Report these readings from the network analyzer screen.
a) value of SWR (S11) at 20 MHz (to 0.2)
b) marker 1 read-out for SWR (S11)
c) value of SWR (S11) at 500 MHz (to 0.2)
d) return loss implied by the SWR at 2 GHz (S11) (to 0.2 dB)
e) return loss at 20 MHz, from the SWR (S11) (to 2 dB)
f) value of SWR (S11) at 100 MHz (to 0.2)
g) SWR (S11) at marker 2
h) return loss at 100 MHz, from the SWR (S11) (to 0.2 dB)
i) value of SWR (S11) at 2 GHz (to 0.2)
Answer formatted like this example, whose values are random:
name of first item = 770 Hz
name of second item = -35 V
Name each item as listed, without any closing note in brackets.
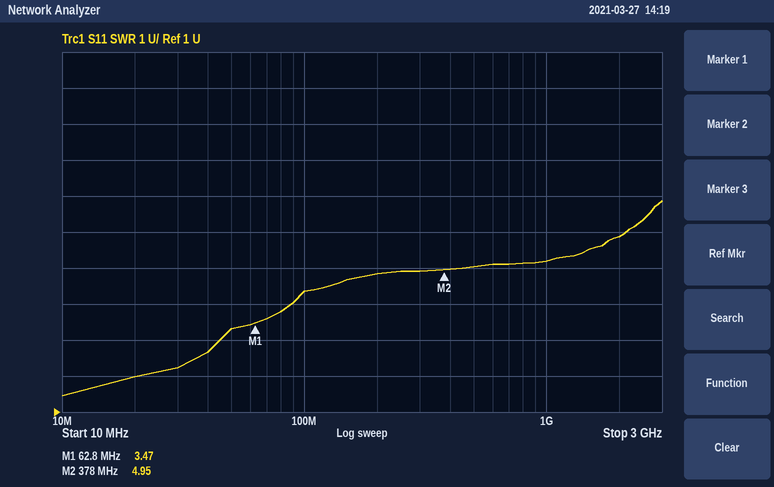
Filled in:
value of SWR (S11) at 20 MHz = 2.0
marker 1 read-out for SWR = 3.47
value of SWR (S11) at 500 MHz = 5.0
return loss implied by the SWR at 2 GHz (S11) = 3.0 dB
return loss at 20 MHz, from the SWR (S11) = 10 dB
value of SWR (S11) at 100 MHz = 4.4
SWR (S11) at marker 2 = 4.95
return loss at 100 MHz, from the SWR (S11) = 4.0 dB
value of SWR (S11) at 2 GHz = 5.8
